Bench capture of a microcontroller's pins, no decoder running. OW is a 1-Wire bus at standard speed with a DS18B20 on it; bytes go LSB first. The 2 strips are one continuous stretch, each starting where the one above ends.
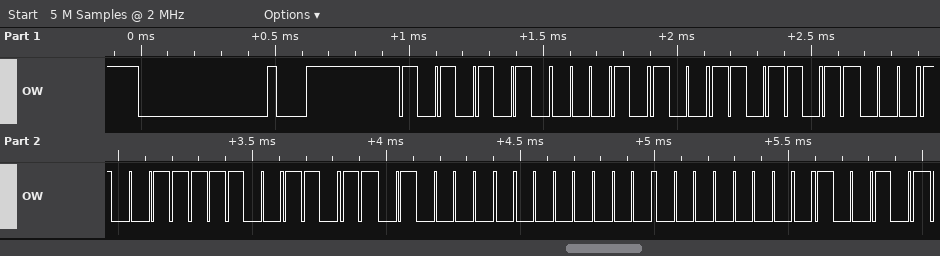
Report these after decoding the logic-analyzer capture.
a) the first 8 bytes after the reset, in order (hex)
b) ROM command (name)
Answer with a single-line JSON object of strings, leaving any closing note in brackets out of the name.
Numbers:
{"the first 8 bytes after the reset, in order": "55 28 DB C8 67 0B 00 00", "ROM command": "Match ROM"}
